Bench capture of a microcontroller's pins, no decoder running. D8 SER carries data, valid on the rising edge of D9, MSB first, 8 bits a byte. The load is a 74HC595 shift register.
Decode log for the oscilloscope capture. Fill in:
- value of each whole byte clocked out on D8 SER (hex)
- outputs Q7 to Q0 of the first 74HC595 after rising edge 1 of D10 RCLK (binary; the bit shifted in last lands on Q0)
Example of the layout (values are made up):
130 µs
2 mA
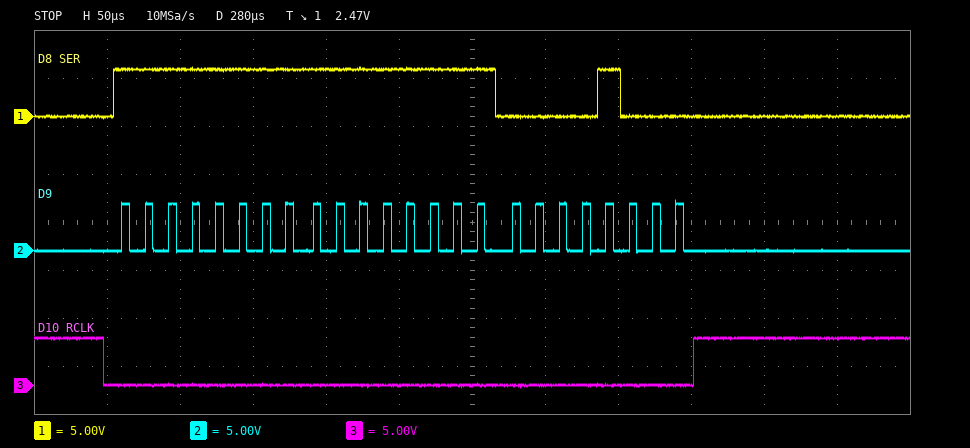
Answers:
0xFF 0xFF 0x08
00001000
